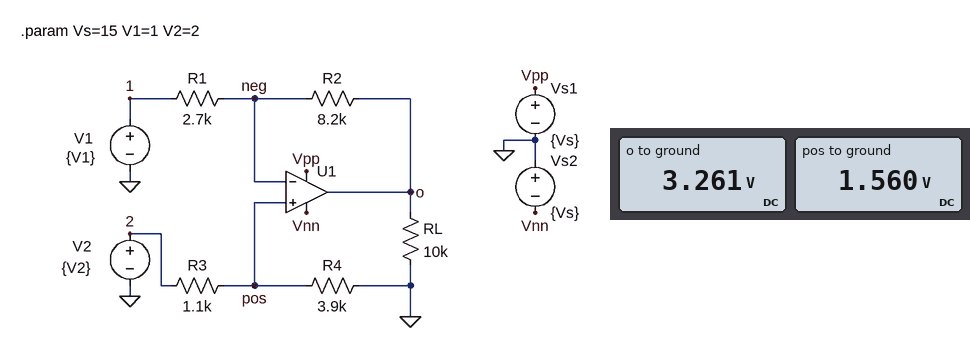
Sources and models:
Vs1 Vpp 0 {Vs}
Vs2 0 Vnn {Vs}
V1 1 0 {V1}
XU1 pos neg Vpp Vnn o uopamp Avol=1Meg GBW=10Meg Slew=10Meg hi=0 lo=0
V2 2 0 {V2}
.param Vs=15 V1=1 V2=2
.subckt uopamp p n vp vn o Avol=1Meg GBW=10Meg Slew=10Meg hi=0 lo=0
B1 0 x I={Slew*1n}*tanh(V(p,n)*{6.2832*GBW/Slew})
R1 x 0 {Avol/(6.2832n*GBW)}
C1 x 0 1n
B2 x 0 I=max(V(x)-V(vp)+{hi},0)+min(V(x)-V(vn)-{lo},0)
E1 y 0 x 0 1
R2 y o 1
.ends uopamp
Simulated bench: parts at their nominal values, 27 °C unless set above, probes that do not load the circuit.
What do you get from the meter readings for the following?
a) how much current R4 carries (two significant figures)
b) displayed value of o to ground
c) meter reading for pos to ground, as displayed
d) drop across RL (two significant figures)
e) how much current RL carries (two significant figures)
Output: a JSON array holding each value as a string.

["400 µA", "3.261 V", "1.560 V", "3.3 V", "330 µA"]
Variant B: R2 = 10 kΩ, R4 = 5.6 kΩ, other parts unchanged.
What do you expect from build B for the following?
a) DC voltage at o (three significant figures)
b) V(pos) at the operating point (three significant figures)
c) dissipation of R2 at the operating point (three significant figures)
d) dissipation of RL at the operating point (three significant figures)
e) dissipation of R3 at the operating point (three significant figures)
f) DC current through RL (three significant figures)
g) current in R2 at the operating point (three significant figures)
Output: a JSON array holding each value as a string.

["4.16 V", "1.67 V", "619 µW", "1.73 mW", "98.0 µW", "416 µA", "249 µA"]
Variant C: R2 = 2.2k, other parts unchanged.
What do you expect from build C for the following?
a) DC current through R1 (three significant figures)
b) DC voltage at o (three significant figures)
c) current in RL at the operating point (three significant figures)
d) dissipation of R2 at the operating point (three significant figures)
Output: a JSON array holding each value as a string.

["207 µA", "2.02 V", "202 µA", "94.6 µW"]
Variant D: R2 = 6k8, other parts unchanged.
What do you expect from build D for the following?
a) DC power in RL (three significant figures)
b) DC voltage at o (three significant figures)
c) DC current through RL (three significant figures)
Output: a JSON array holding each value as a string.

["882 µW", "2.97 V", "297 µA"]
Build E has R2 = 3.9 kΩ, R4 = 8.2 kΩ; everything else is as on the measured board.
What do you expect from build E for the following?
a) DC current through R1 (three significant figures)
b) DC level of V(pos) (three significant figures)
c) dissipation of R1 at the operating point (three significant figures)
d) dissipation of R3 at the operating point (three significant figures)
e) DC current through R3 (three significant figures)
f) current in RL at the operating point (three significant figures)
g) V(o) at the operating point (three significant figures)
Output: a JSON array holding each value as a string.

["283 µA", "1.76 V", "216 µW", "50.9 µW", "215 µA", "287 µA", "2.87 V"]
